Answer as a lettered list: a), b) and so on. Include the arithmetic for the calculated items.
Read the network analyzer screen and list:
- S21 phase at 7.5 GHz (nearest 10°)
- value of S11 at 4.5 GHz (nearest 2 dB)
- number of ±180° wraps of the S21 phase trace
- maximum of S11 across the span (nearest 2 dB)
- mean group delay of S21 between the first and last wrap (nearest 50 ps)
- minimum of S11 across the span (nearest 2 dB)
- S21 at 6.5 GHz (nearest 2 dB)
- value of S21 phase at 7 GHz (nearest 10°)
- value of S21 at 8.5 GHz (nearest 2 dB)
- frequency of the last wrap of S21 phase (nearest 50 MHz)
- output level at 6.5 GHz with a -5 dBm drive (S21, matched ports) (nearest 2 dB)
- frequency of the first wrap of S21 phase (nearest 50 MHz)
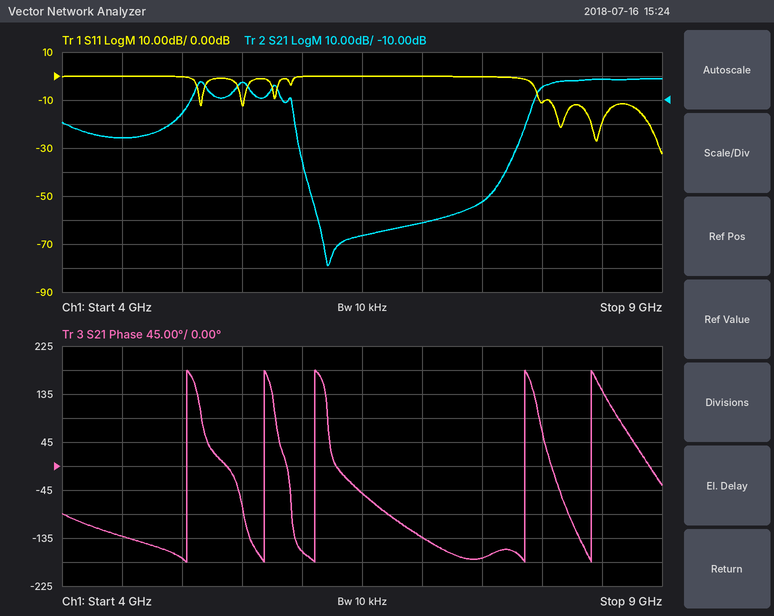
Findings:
a) -170°
b) 0 dB
c) 5
d) 0 dB
e) 4 cycles / (8.40 GHz − 5.05 GHz) ≈ 1.19 ns, so 1.20 ns to the nearest 50 ps
f) -32 dB
g) -66 dB
h) -130°
i) -2 dB
j) 8.40 GHz
k) -5 dBm + (-66 dB) = -72 dBm
l) 5.05 GHz
